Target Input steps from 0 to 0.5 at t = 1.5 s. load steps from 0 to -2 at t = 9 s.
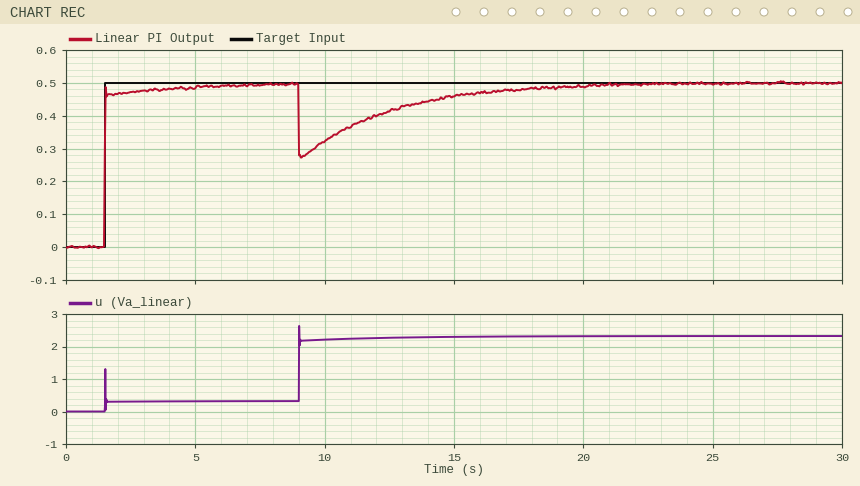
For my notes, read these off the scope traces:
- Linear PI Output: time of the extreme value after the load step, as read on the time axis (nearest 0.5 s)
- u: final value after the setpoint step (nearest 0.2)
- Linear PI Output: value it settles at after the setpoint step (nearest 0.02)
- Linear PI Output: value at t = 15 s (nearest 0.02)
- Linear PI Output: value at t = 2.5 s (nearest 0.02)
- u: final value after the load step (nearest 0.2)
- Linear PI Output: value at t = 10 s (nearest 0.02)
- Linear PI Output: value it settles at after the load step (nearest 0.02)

9.0 s
0.4
0.50
0.46
0.48
2.4
0.32
0.50
